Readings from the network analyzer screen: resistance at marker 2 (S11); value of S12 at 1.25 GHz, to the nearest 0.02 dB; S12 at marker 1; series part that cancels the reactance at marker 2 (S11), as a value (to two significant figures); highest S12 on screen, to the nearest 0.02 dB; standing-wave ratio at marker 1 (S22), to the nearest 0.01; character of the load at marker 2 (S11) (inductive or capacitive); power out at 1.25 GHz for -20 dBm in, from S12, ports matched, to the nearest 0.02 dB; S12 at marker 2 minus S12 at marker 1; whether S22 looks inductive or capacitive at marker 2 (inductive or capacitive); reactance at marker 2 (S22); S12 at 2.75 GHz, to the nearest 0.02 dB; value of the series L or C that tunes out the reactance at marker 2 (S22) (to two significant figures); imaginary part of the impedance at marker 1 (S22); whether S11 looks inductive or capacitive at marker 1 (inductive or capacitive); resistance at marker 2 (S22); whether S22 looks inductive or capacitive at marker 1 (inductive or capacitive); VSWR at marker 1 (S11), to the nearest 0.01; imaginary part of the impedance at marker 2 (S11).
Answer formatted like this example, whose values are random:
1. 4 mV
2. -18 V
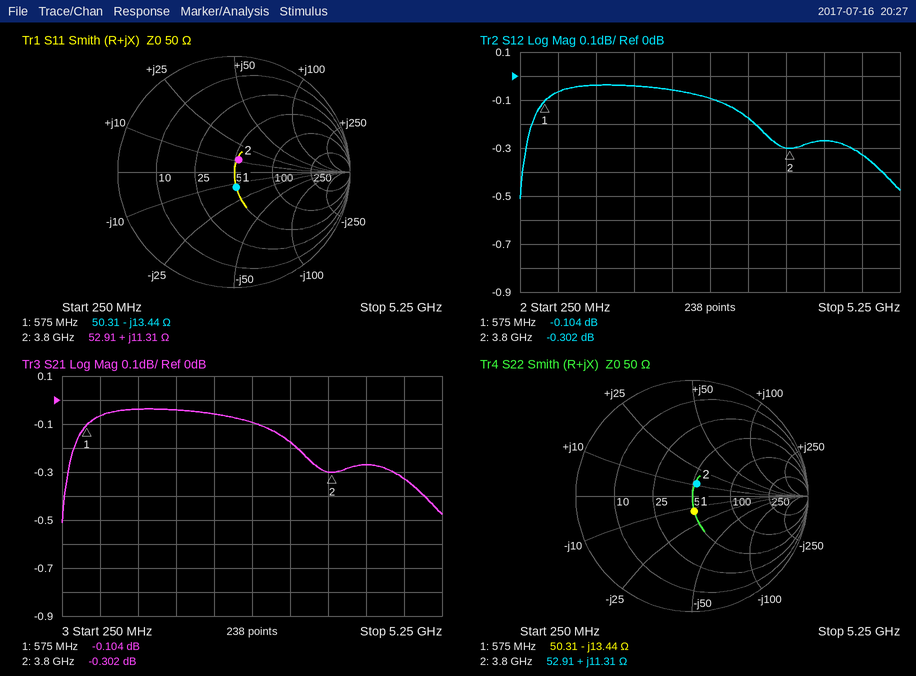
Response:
1. 52.91 Ω
2. -0.04 dB
3. -0.104 dB
4. 3.7 pF
5. -0.04 dB
6. 1.31
7. inductive
8. -20.04 dBm
9. -0.198 dB
10. inductive
11. +11.31 Ω
12. -0.10 dB
13. 3.7 pF
14. -13.44 Ω
15. capacitive
16. 52.91 Ω
17. capacitive
18. 1.31
19. +11.31 Ω
